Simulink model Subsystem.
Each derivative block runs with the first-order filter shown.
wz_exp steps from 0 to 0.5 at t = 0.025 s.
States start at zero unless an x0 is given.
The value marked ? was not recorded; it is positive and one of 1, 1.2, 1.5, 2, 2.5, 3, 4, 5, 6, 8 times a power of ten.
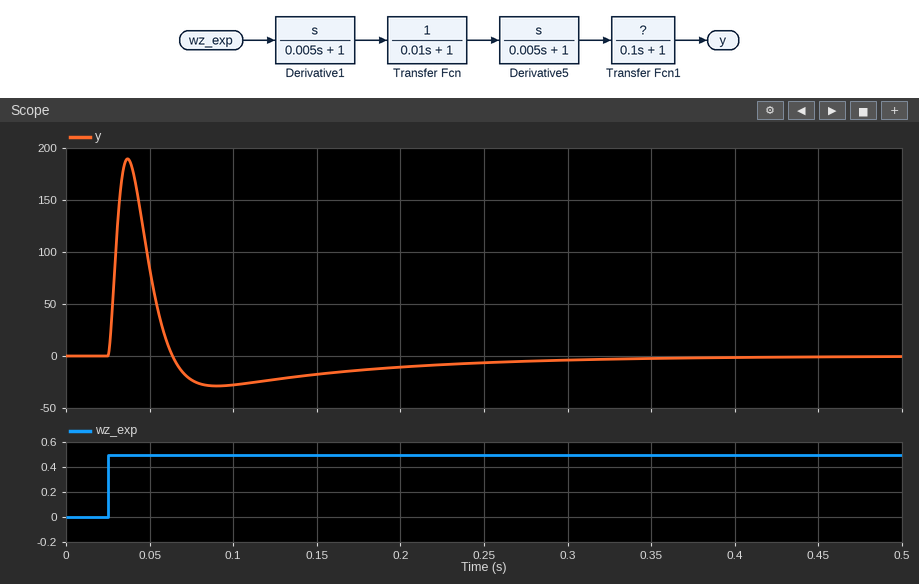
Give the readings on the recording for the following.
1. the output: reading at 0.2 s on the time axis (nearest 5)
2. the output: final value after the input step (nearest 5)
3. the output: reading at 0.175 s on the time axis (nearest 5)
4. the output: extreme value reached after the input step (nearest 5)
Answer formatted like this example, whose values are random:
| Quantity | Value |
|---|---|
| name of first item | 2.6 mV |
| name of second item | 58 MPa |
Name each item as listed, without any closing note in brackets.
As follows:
| Quantity | Value |
|---|---|
| the output: reading at 0.2 s on the time axis | -10 |
| the output: final value after the input step | 0 |
| the output: reading at 0.175 s on the time axis | -15 |
| the output: extreme value reached after the input step | 190 |
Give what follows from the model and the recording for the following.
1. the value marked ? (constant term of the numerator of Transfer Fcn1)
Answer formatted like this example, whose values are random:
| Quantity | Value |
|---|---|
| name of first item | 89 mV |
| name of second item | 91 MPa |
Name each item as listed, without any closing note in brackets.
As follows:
| Quantity | Value |
|---|---|
| the value marked ? | 1 |
